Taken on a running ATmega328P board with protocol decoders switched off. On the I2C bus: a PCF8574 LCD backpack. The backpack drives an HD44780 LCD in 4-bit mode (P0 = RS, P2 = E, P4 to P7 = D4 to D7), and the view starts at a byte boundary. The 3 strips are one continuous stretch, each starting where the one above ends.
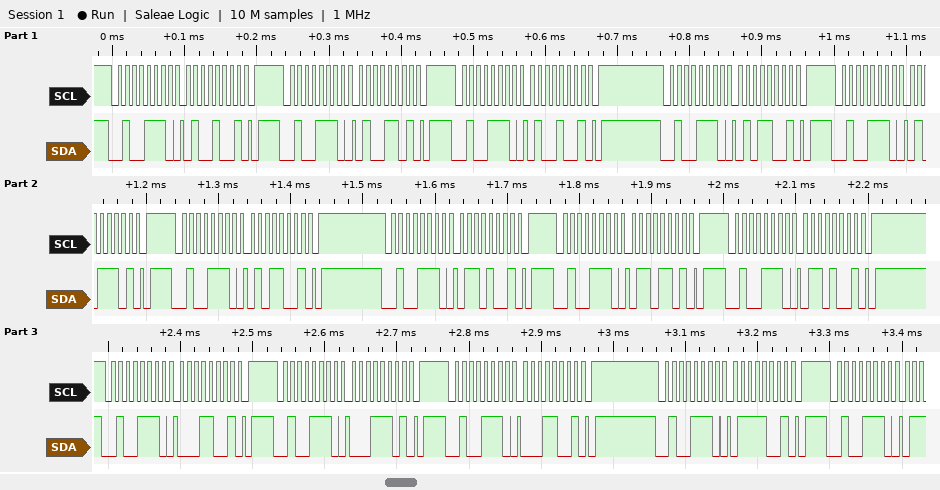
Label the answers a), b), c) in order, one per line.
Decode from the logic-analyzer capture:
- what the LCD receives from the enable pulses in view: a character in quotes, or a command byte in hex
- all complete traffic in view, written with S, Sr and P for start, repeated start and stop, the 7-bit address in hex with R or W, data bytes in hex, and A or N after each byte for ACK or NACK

a) 'E' 'a'
b) S 27W A 49 A P S 27W A 4D A P S 27W A 49 A P S 27W A 59 A P S 27W A 5D A P S 27W A 59 A P S 27W A 69 A P S 27W A 6D A P S 27W A 69 A P S 27W A 19 A P S 27W A 1D A P S 27W A 19 A P S 27W A 79 A P S 27W A
